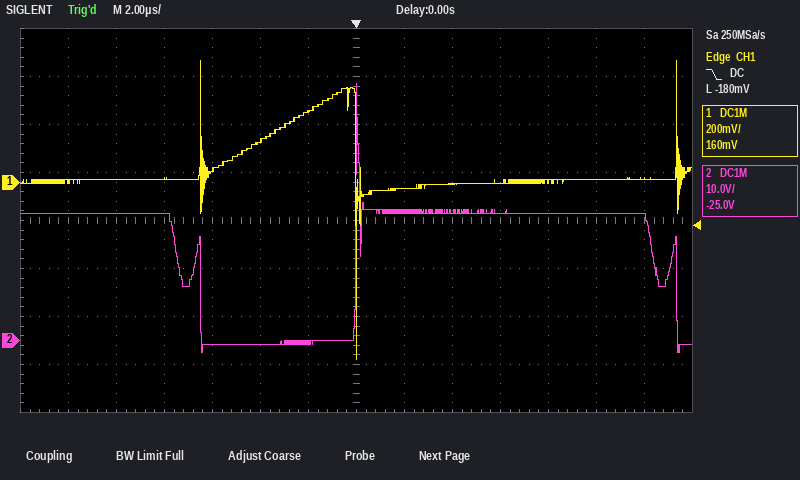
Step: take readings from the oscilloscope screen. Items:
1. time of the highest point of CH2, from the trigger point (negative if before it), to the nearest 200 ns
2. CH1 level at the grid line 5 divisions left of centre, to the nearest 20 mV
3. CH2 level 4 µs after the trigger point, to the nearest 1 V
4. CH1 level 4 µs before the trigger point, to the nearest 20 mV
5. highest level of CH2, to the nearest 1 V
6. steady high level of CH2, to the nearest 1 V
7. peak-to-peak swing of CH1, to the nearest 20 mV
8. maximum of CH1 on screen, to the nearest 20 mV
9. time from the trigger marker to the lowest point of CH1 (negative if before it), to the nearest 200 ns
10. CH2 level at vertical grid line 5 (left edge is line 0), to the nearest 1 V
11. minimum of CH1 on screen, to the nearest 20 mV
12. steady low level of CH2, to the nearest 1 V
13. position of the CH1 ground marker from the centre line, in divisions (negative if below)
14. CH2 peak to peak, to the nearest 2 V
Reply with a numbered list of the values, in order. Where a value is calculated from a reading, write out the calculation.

1. 0.0 µs
2. 20 mV
3. 27 V
4. 180 mV
5. 54 V
6. 26 V
7. 500 mV − (-740 mV) = 1.24 V
8. 500 mV
9. 0.0 µs
10. -1 V
11. -740 mV
12. -1 V
13. +0.8 div
14. 56 V
